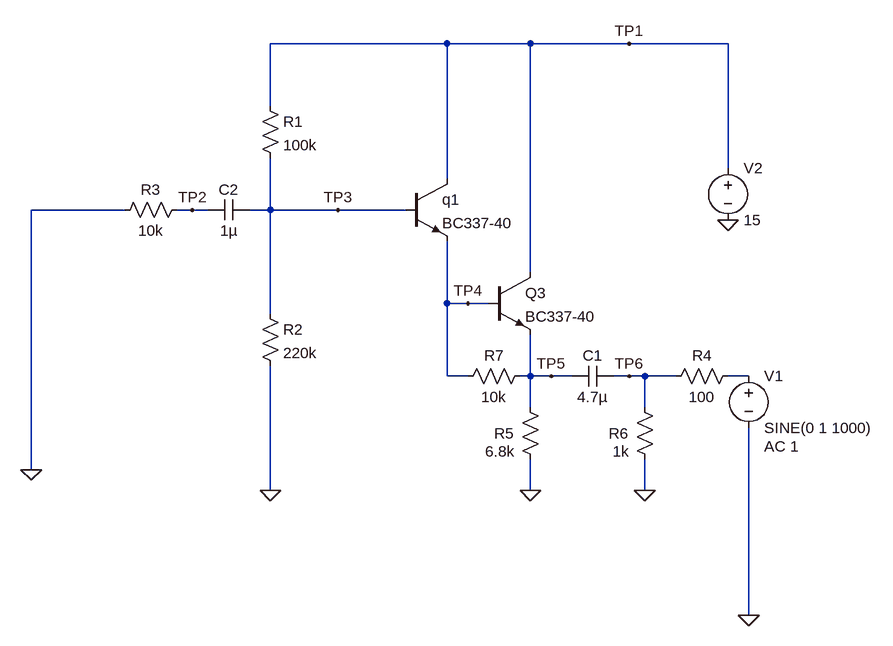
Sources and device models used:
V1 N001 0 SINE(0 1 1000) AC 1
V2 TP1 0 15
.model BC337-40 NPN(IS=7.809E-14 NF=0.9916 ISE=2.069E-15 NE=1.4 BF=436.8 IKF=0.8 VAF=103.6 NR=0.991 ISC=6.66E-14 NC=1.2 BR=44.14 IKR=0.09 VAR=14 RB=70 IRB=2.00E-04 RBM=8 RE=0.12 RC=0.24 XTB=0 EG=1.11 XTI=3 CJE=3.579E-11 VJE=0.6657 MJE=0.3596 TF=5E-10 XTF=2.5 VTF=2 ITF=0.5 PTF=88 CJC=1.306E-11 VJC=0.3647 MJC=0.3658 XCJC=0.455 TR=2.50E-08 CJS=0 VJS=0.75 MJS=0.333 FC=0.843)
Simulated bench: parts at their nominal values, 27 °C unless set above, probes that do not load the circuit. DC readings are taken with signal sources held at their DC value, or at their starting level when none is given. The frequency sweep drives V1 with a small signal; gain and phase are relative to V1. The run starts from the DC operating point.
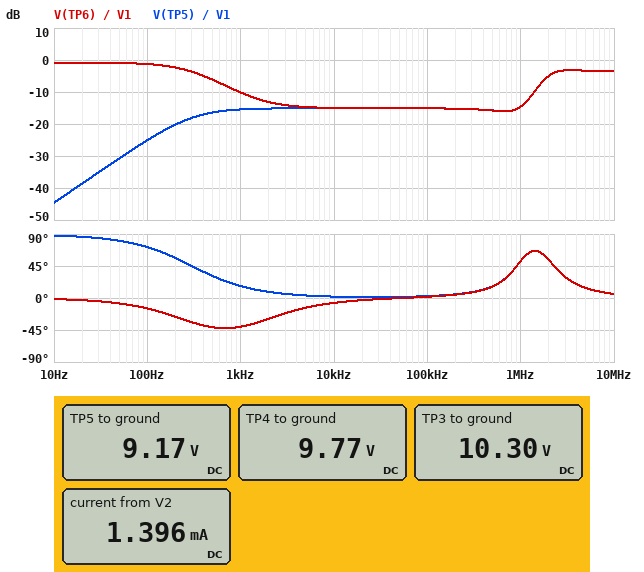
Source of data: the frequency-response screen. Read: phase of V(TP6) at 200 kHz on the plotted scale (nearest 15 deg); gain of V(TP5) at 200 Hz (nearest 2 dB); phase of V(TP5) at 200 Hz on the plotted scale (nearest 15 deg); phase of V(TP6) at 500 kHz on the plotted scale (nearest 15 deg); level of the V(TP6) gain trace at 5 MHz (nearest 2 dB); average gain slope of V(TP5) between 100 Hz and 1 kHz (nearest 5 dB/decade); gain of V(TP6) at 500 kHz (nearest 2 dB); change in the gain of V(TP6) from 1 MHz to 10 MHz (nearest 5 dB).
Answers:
0 deg
-20 dB
60 deg
15 deg
-4 dB
10 dB/decade
-16 dB
10 dB
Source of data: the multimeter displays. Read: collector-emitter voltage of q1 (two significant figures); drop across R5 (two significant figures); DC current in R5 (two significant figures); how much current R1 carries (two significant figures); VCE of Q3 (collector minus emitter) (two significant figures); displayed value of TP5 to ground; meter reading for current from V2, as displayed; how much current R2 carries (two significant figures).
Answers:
5.2 V
9.2 V
1.3 mA
47 µA
5.8 V
9.17 V
1.396 mA
47 µA
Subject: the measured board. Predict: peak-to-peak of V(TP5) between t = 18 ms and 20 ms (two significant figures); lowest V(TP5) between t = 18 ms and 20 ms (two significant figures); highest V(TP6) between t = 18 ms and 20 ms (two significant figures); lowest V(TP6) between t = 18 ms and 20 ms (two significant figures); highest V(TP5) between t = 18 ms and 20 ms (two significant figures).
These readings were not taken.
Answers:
1.3 V
9.1 V
770 mV
-580 mV
10 V
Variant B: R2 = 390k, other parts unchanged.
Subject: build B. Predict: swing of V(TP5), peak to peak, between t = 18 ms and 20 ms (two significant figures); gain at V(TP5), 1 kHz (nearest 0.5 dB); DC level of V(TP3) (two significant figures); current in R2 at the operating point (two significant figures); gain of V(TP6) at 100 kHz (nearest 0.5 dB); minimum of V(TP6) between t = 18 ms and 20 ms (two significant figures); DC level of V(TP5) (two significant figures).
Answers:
1.2 V
-16.5 dB
12 V
31 µA
-16.0 dB
-550 mV
11 V
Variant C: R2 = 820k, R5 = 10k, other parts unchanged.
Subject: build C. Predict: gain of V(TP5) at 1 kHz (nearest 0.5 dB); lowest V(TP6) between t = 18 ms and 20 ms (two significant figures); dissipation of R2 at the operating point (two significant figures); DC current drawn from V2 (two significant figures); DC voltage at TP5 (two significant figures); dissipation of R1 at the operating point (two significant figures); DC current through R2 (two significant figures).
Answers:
-14.5 dB
-590 mV
220 µW
1.2 mA
12 V
27 µW
16 µA
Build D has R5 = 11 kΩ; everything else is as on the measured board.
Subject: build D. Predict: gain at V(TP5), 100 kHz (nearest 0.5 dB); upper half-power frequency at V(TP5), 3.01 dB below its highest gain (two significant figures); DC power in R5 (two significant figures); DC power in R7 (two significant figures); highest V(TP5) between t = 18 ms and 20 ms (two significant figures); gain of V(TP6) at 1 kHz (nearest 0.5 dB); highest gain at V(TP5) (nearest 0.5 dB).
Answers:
-12.0 dB
320 MHz
7.7 mW
35 µW
11 V
-9.5 dB
-2.5 dB
